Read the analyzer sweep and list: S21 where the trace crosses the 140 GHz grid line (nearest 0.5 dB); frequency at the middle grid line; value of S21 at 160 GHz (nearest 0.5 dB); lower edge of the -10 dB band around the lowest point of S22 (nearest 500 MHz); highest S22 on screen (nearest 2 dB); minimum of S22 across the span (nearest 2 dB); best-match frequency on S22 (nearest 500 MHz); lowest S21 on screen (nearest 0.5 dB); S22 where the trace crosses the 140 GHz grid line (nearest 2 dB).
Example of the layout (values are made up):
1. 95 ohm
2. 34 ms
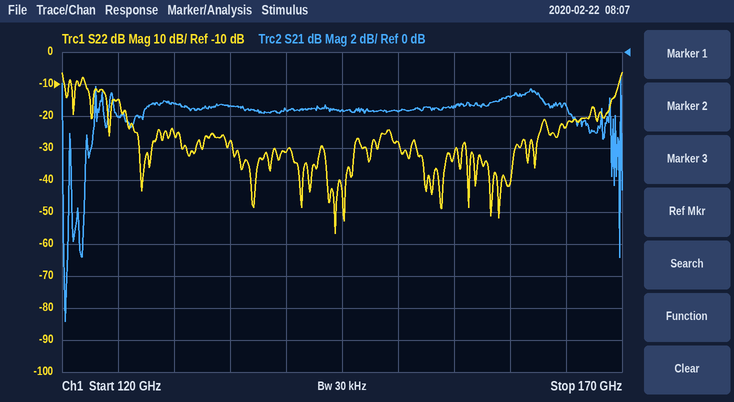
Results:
1. -3.5 dB
2. 145 GHz
3. -3.0 dB
4. 122.0 GHz
5. -6 dB
6. -56 dB
7. 144.5 GHz
8. -17.0 dB
9. -32 dB
